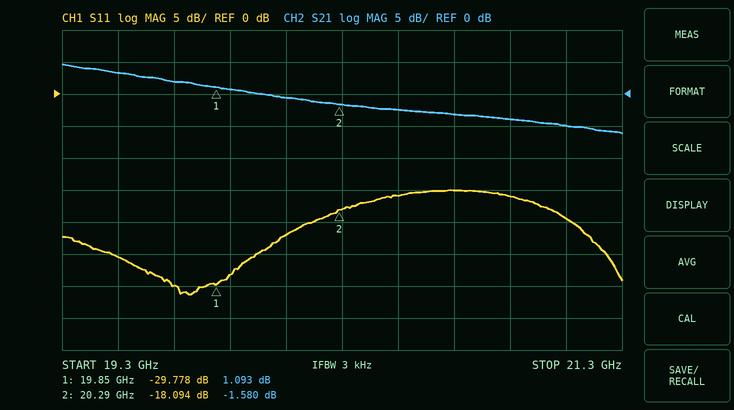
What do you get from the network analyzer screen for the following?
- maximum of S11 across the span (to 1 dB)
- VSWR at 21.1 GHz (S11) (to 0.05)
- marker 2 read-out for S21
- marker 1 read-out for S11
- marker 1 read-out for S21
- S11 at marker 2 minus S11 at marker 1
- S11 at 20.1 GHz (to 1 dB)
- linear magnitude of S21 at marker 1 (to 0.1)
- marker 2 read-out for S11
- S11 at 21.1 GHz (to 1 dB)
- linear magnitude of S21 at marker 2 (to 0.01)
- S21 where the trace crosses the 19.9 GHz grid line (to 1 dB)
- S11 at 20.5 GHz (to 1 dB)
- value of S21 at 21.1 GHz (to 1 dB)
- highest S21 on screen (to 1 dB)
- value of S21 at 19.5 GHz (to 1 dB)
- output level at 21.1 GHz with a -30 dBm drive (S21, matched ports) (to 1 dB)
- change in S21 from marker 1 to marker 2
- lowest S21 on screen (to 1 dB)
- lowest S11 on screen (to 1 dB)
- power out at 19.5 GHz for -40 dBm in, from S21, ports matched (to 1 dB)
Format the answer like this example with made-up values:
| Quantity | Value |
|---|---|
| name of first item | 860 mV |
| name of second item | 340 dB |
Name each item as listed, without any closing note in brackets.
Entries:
| Quantity | Value |
|---|---|
| maximum of S11 across the span | -15 dB |
| VSWR at 21.1 GHz (S11) | 1.25 |
| marker 2 read-out for S21 | -1.580 dB |
| marker 1 read-out for S11 | -29.778 dB |
| marker 1 read-out for S21 | 1.093 dB |
| S11 at marker 2 minus S11 at marker 1 | 11.684 dB |
| S11 at 20.1 GHz | -22 dB |
| linear magnitude of S21 at marker 1 | 1.1 |
| marker 2 read-out for S11 | -18.094 dB |
| S11 at 21.1 GHz | -19 dB |
| linear magnitude of S21 at marker 2 | 0.83 |
| S21 where the trace crosses the 19.9 GHz grid line | 1 dB |
| S11 at 20.5 GHz | -16 dB |
| value of S21 at 21.1 GHz | -5 dB |
| highest S21 on screen | 5 dB |
| value of S21 at 19.5 GHz | 3 dB |
| output level at 21.1 GHz with a -30 dBm drive (S21, matched ports) | -35 dBm |
| change in S21 from marker 1 to marker 2 | -2.673 dB |
| lowest S21 on screen | -6 dB |
| lowest S11 on screen | -31 dB |
| power out at 19.5 GHz for -40 dBm in, from S21, ports matched | -37 dBm |
